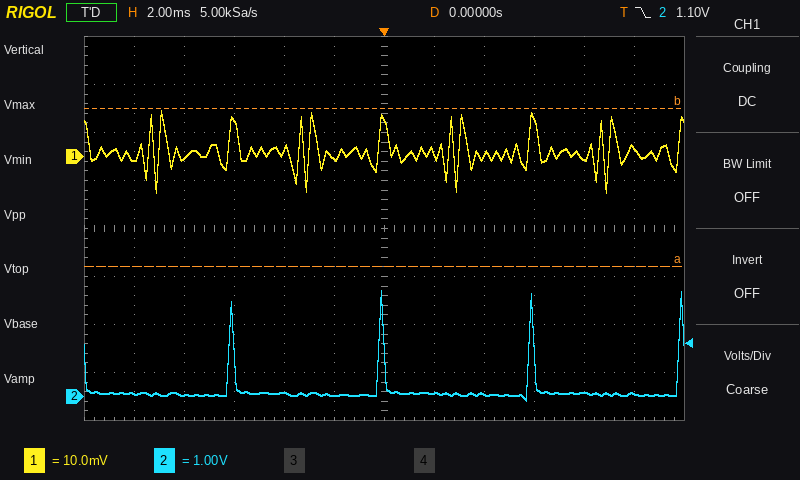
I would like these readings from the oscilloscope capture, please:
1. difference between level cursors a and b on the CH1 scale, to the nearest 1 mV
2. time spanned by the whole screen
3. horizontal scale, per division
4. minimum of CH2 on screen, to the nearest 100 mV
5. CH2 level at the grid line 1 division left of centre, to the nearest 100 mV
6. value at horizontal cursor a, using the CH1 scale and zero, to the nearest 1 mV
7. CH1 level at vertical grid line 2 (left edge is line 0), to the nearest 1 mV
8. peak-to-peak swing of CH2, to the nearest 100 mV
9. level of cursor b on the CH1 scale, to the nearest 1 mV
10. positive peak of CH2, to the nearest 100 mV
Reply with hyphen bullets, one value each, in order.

- 33 mV
- 24 ms
- 2 ms
- -100 mV
- 0.0 V
- -23 mV
- 0 mV
- 2.3 V
- 10 mV
- 2.2 V
